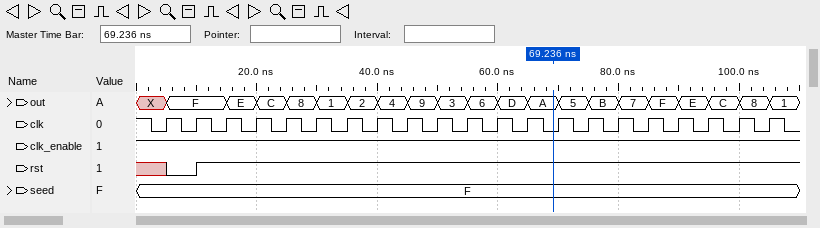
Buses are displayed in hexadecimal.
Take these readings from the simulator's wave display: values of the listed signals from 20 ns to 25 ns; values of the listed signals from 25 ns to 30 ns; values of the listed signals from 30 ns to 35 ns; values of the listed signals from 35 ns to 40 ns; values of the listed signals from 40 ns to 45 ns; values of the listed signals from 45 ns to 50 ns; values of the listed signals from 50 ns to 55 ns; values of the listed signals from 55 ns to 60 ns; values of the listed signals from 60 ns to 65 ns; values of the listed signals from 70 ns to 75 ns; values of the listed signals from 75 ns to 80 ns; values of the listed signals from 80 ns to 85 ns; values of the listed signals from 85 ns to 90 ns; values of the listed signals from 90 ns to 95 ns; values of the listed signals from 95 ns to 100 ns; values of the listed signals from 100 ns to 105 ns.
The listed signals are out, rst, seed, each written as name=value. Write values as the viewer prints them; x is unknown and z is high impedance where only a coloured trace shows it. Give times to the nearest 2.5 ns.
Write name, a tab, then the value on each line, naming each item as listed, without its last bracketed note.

values of the listed signals from 20 ns to 25 ns	out=C, rst=1, seed=F
values of the listed signals from 25 ns to 30 ns	out=8, rst=1, seed=F
values of the listed signals from 30 ns to 35 ns	out=1, rst=1, seed=F
values of the listed signals from 35 ns to 40 ns	out=2, rst=1, seed=F
values of the listed signals from 40 ns to 45 ns	out=4, rst=1, seed=F
values of the listed signals from 45 ns to 50 ns	out=9, rst=1, seed=F
values of the listed signals from 50 ns to 55 ns	out=3, rst=1, seed=F
values of the listed signals from 55 ns to 60 ns	out=6, rst=1, seed=F
values of the listed signals from 60 ns to 65 ns	out=D, rst=1, seed=F
values of the listed signals from 70 ns to 75 ns	out=5, rst=1, seed=F
values of the listed signals from 75 ns to 80 ns	out=B, rst=1, seed=F
values of the listed signals from 80 ns to 85 ns	out=7, rst=1, seed=F
values of the listed signals from 85 ns to 90 ns	out=F, rst=1, seed=F
values of the listed signals from 90 ns to 95 ns	out=E, rst=1, seed=F
values of the listed signals from 95 ns to 100 ns	out=C, rst=1, seed=F
values of the listed signals from 100 ns to 105 ns	out=8, rst=1, seed=F
